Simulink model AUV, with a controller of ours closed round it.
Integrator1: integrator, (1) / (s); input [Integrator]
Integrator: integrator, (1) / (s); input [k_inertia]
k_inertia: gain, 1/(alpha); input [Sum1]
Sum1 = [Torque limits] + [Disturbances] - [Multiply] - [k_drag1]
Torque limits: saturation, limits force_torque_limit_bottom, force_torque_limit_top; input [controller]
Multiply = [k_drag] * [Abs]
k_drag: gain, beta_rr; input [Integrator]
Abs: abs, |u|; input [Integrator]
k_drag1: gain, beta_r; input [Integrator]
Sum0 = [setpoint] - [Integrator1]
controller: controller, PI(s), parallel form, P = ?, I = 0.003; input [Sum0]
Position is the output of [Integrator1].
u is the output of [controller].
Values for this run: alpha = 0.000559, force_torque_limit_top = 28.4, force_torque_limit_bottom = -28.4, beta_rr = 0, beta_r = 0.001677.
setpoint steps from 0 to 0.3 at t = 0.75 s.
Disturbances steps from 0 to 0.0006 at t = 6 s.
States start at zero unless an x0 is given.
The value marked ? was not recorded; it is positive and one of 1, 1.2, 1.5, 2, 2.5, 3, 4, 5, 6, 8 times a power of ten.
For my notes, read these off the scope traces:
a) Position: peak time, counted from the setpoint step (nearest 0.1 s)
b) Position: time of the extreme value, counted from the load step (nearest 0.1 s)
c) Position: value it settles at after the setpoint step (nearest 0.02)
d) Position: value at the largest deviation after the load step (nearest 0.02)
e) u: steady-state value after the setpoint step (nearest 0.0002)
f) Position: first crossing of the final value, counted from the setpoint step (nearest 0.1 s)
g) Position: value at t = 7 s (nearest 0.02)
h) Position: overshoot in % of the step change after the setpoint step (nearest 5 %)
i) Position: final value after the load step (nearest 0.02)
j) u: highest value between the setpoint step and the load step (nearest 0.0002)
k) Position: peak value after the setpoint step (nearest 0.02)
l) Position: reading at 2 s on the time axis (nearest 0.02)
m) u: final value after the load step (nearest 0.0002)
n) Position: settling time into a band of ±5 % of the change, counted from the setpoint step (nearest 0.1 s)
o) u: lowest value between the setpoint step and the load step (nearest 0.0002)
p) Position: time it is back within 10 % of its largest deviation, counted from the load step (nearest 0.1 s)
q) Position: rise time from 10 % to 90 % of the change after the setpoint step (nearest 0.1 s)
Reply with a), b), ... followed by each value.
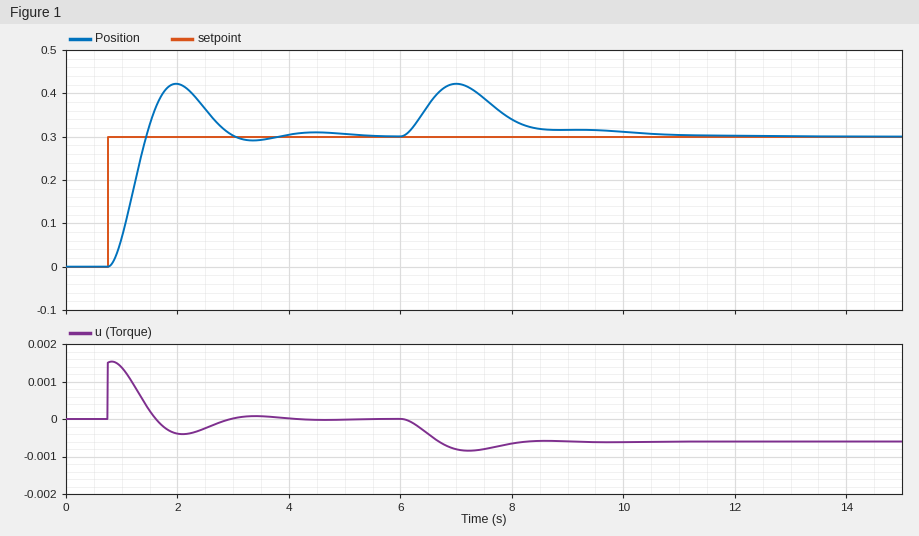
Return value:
a) 1.2 s
b) 1.0 s
c) 0.30
d) 0.42
e) 0.0000
f) 0.7 s
g) 0.42
h) 40 %
i) 0.30
j) 0.0016
k) 0.42
l) 0.42
m) -0.0006
n) 2.1 s
o) -0.0004
p) 3.9 s
q) 0.5 s
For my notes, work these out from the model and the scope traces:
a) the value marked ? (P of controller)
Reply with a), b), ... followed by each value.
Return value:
a) 0.005
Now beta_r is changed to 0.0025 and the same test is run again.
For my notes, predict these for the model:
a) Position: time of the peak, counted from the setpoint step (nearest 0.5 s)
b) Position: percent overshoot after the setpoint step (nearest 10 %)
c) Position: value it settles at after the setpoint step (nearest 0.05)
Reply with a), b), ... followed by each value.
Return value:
a) 1.5 s
b) 30 %
c) 0.30
